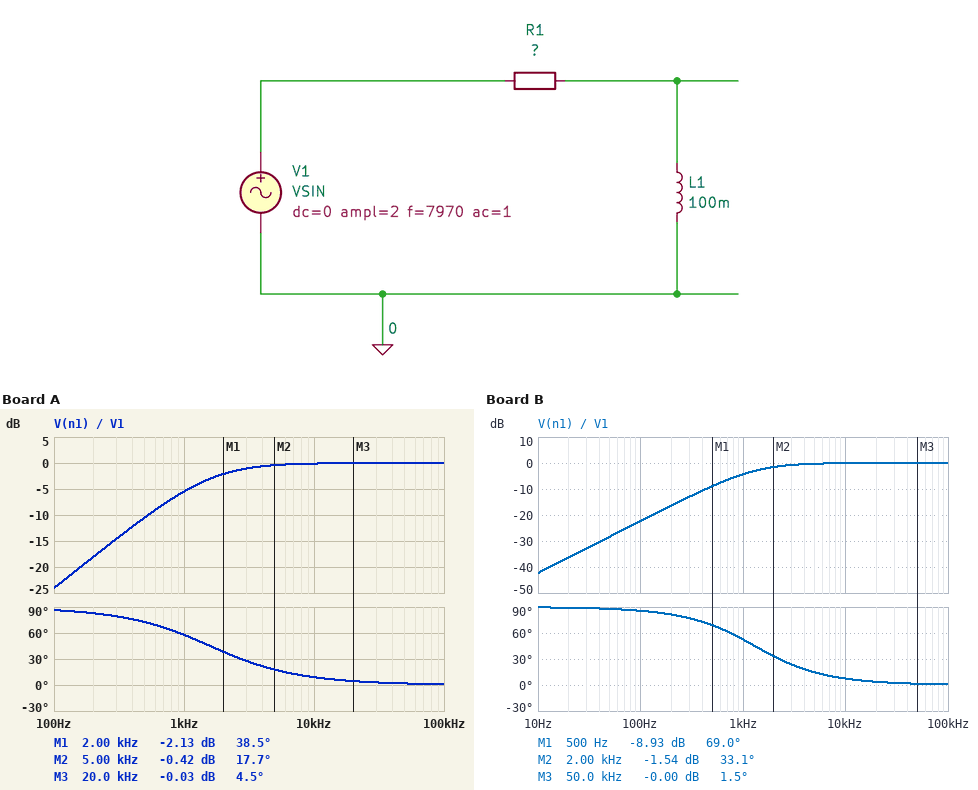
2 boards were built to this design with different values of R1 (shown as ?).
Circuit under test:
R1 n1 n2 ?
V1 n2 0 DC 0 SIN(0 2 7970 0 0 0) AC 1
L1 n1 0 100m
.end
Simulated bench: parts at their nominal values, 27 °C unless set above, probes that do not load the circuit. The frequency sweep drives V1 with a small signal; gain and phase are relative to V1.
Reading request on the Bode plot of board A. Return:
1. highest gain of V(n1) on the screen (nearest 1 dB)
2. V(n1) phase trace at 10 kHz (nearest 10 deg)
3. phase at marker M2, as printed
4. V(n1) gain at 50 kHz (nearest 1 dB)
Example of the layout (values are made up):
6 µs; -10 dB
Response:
0 dB; 10 deg; 17.7 deg; 0 dB
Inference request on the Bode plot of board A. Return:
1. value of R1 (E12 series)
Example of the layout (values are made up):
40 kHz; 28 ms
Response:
1 kΩ
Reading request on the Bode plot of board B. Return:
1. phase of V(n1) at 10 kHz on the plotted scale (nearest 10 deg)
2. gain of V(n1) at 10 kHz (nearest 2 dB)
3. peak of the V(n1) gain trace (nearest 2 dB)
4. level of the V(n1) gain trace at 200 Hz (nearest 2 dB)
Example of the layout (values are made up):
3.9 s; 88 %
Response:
10 deg; 0 dB; 0 dB; -16 dB
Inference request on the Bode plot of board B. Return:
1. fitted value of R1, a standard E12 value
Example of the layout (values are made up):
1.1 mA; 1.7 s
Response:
820 Ω
